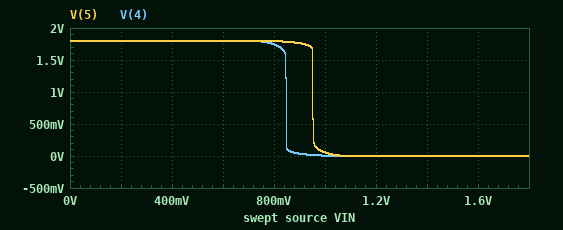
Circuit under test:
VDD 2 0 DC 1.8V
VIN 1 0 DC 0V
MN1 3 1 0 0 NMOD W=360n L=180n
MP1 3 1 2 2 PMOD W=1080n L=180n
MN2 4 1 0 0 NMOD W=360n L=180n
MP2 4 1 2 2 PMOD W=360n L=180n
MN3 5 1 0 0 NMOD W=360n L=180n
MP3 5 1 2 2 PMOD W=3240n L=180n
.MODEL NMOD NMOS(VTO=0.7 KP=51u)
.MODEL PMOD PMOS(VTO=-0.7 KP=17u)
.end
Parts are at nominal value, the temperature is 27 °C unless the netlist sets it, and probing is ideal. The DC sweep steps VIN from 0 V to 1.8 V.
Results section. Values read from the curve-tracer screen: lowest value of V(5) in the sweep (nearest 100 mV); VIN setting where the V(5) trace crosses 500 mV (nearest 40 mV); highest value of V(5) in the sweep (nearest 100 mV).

0 V
960 mV
1.8 V
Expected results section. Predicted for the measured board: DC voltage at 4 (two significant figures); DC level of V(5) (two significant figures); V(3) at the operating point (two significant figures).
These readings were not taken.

1.8 V
1.8 V
1.8 V
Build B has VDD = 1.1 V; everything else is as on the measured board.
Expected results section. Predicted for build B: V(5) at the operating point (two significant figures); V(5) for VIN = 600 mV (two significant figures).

1.1 V
550 mV
